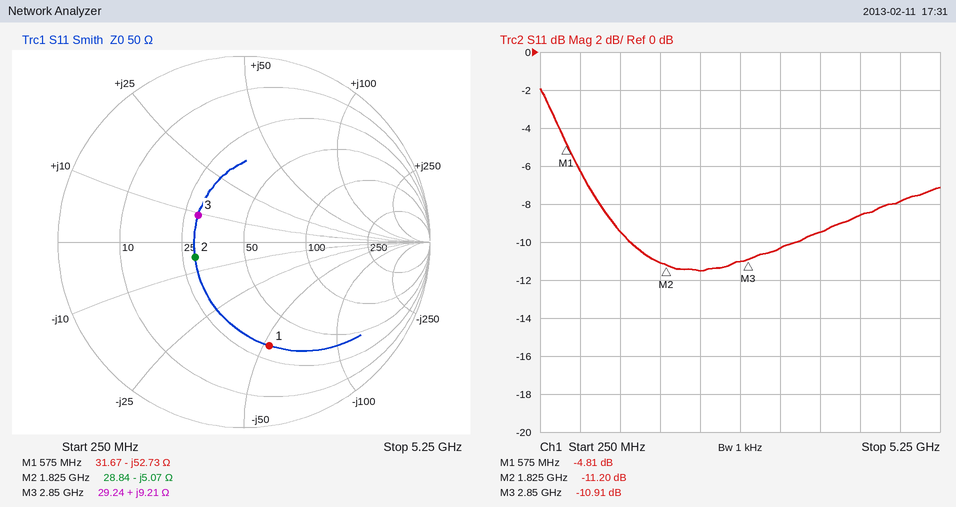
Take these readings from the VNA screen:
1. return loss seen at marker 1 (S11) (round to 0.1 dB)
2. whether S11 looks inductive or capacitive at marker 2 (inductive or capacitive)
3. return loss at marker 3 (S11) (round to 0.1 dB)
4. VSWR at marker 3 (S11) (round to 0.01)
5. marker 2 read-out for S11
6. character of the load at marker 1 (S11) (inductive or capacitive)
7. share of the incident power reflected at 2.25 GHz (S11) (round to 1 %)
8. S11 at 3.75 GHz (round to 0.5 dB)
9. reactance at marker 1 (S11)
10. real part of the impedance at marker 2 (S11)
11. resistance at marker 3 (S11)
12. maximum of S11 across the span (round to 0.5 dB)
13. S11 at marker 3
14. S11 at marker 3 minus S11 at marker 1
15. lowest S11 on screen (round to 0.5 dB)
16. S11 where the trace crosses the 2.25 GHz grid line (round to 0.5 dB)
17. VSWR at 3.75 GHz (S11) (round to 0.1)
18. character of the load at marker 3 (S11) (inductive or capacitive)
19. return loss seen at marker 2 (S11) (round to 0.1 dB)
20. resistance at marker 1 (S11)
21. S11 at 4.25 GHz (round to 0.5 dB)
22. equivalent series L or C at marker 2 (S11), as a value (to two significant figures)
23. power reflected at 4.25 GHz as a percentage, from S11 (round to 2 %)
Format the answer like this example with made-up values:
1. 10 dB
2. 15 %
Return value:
1. 4.8 dB
2. capacitive
3. 10.9 dB
4. 1.80
5. -11.20 dB
6. capacitive
7. 7 %
8. -9.5 dB
9. -52.73 Ω
10. 28.84 Ω
11. 29.24 Ω
12. -2.0 dB
13. -10.91 dB
14. -6.10 dB
15. -11.5 dB
16. -11.5 dB
17. 2.0
18. inductive
19. 11.2 dB
20. 31.67 Ω
21. -8.5 dB
22. 17 pF
23. 14 %
